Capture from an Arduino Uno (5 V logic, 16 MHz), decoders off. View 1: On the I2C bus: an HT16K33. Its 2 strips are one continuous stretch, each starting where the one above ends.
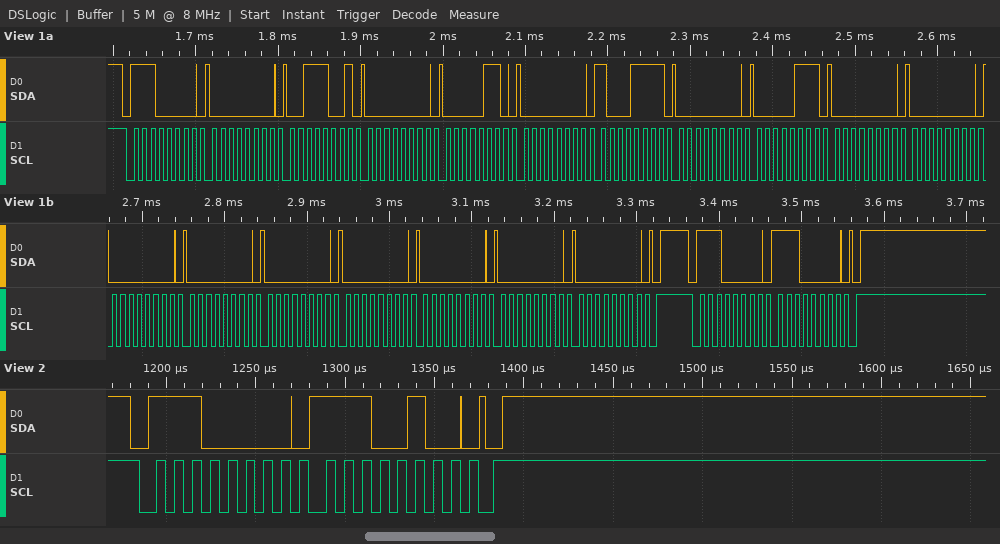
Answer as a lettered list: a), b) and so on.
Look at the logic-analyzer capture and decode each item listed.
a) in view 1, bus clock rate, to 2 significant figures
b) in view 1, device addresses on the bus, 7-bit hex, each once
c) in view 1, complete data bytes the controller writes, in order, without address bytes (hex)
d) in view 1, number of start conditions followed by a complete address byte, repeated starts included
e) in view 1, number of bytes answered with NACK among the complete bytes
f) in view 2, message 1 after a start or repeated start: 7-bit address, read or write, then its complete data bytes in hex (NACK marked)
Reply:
a) 100 kHz
b) 0x70
c) 00 39 00 06 00 8F 00 07 00 00 00 00 00 00 00 00 00 E0
d) 2
e) 0
f) 0x70 write: E4
